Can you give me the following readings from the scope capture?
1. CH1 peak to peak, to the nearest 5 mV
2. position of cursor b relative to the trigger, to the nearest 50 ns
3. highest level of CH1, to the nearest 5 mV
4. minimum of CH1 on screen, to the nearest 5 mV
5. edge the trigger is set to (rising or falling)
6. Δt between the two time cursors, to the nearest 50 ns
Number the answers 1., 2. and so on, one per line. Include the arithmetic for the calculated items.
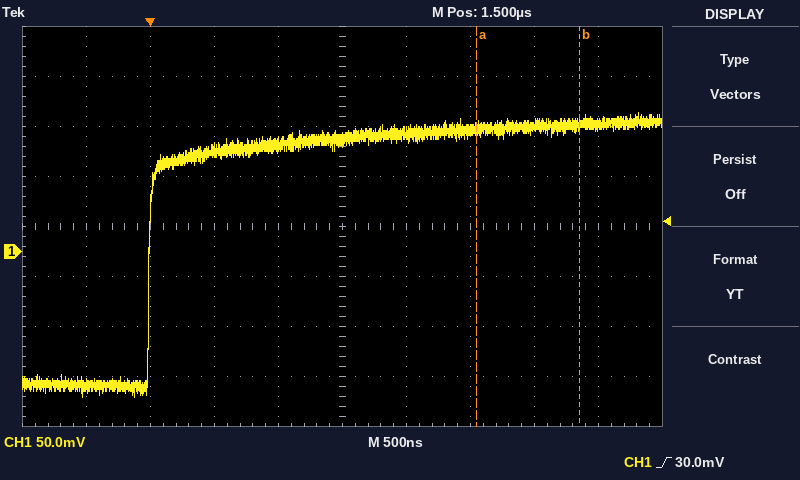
1. 140 mV − (-145 mV) = 285 mV
2. +3.35 µs
3. 140 mV
4. -145 mV
5. rising
6. 800 ns
